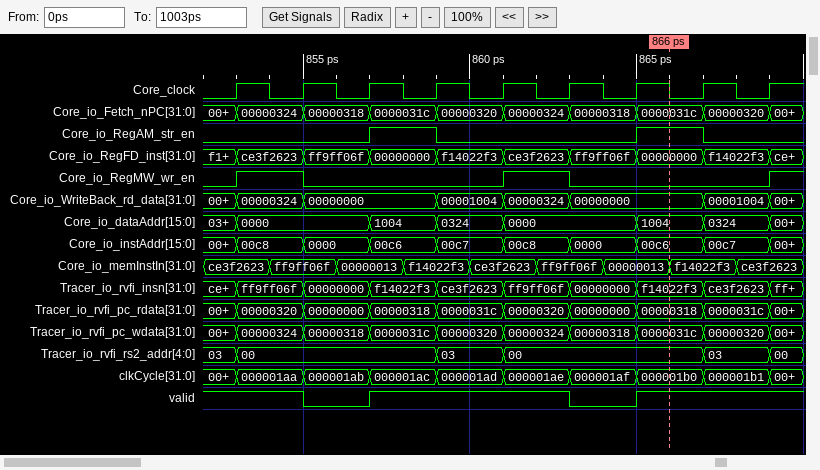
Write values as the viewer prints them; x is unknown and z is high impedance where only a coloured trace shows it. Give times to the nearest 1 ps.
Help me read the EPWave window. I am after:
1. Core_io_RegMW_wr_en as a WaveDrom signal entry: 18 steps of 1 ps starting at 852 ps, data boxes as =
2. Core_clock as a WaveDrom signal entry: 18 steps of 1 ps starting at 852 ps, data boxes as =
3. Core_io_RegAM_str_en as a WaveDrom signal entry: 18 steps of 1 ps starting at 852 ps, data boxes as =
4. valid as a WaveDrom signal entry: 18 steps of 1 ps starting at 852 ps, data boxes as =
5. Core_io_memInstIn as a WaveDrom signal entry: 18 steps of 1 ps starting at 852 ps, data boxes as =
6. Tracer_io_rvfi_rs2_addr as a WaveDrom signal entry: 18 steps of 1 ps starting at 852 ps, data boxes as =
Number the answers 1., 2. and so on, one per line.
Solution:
1. {name: 'Core_io_RegMW_wr_en', wave: '01.0.....1.0.....1'}
2. {name: 'Core_clock', wave: '010101010101010101'}
3. {name: 'Core_io_RegAM_str_en', wave: '0....1.0.....1.0..'}
4. {name: 'valid', wave: '1..0.1.....0.1....'}
5. {name: 'Core_io_memInstIn', wave: '=.=.=.=.=.=.=.=.=.', data: 'ce3f2623 ff9ff06f 00000013 f14022f3 ce3f2623 ff9ff06f 00000013 f14022f3 ce3f2623'}
6. {name: 'Tracer_io_rvfi_rs2_addr', wave: '==.....=.=.....=.=', data: '03 00 03 00 03 00'}
